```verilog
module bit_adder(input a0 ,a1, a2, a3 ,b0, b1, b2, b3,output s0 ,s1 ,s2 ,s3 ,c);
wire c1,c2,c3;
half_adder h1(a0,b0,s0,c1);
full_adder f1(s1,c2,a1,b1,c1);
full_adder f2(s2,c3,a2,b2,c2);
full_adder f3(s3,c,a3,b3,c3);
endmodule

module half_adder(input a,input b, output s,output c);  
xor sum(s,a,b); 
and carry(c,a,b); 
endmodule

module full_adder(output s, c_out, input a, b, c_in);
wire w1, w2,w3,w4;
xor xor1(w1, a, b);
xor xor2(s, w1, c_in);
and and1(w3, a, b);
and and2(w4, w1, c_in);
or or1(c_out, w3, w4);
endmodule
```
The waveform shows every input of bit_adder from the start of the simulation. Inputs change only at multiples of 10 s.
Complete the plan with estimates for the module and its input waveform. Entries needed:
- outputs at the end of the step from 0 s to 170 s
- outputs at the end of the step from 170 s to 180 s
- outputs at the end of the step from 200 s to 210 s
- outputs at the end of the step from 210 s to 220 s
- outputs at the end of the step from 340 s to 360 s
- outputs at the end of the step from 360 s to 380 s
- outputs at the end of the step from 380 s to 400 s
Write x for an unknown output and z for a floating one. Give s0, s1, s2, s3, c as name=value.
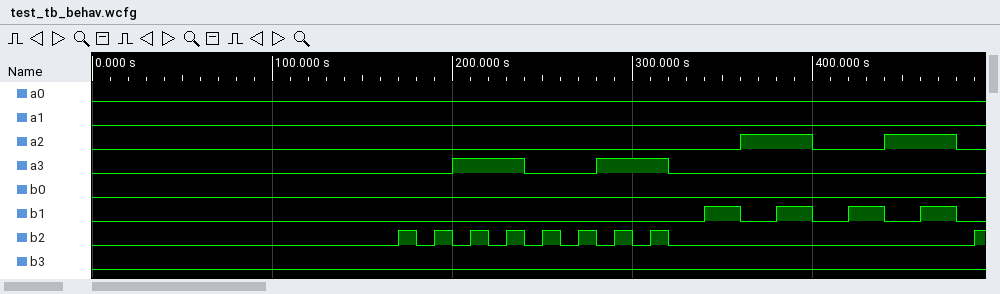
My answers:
s0=0, s1=0, s2=0, s3=0, c=0
s0=0, s1=0, s2=1, s3=0, c=0
s0=0, s1=0, s2=0, s3=1, c=0
s0=0, s1=0, s2=1, s3=1, c=0
s0=0, s1=1, s2=0, s3=0, c=0
s0=0, s1=0, s2=1, s3=0, c=0
s0=0, s1=1, s2=1, s3=0, c=0
